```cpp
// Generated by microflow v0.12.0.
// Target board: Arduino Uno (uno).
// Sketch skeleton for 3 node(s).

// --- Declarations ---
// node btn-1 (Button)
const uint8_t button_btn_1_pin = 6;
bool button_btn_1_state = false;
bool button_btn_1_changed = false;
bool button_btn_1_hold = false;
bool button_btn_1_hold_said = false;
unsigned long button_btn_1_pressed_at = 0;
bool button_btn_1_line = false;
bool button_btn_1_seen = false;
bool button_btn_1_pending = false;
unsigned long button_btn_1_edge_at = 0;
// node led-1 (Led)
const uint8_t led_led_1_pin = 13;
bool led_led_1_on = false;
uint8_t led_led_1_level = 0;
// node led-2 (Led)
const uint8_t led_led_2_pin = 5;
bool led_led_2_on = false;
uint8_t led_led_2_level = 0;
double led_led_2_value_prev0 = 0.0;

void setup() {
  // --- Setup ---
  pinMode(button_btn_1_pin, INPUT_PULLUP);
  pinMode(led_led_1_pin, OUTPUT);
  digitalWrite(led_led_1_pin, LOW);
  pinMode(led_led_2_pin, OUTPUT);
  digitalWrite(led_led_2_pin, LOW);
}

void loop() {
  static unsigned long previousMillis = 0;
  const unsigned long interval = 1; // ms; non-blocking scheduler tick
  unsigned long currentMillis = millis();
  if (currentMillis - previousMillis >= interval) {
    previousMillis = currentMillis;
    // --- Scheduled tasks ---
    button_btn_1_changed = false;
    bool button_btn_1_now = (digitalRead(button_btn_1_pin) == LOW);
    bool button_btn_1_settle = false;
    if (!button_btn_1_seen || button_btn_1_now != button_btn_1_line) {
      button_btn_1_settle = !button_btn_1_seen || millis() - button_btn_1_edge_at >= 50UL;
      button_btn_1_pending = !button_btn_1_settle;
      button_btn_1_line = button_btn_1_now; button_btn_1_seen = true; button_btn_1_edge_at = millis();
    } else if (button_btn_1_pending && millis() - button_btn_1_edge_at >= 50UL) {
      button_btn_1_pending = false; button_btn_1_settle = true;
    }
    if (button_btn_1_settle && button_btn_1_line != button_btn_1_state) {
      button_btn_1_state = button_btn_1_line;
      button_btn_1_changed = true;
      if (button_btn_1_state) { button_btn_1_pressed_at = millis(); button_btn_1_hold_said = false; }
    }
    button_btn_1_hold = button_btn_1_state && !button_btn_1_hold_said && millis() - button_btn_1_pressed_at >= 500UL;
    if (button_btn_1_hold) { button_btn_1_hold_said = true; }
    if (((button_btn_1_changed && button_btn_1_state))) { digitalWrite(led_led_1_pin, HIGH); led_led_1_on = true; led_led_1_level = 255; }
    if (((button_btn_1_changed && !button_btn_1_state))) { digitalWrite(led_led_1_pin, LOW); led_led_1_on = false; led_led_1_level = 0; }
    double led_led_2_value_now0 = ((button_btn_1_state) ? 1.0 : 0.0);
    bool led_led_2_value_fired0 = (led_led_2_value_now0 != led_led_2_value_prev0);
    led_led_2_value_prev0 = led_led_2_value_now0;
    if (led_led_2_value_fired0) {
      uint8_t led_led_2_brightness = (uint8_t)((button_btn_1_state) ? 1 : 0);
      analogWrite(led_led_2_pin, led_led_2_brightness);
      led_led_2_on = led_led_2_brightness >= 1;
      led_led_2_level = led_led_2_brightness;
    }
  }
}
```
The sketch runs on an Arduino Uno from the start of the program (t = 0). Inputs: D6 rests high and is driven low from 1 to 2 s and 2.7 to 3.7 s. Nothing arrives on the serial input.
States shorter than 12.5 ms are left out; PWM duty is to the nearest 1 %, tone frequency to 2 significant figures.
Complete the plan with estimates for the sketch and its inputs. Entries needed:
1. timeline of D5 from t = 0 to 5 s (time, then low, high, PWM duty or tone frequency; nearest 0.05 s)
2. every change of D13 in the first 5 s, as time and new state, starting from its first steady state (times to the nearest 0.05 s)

0 s low; 1 s PWM 1 %; 2 s low; 2.7 s PWM 1 %; 3.7 s low
0 s low; 1 s high; 2 s low; 2.7 s high; 3.7 s low
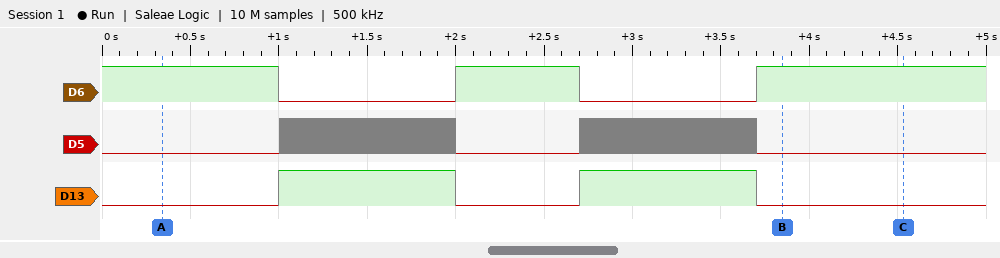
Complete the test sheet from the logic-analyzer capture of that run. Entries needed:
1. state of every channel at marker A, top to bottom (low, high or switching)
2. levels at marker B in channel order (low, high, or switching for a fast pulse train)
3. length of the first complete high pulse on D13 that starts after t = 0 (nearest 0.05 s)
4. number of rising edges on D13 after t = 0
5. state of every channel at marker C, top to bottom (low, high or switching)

D6 high, D5 low, D13 low
D6 high, D5 low, D13 low
1.00 s
2
D6 high, D5 low, D13 low
